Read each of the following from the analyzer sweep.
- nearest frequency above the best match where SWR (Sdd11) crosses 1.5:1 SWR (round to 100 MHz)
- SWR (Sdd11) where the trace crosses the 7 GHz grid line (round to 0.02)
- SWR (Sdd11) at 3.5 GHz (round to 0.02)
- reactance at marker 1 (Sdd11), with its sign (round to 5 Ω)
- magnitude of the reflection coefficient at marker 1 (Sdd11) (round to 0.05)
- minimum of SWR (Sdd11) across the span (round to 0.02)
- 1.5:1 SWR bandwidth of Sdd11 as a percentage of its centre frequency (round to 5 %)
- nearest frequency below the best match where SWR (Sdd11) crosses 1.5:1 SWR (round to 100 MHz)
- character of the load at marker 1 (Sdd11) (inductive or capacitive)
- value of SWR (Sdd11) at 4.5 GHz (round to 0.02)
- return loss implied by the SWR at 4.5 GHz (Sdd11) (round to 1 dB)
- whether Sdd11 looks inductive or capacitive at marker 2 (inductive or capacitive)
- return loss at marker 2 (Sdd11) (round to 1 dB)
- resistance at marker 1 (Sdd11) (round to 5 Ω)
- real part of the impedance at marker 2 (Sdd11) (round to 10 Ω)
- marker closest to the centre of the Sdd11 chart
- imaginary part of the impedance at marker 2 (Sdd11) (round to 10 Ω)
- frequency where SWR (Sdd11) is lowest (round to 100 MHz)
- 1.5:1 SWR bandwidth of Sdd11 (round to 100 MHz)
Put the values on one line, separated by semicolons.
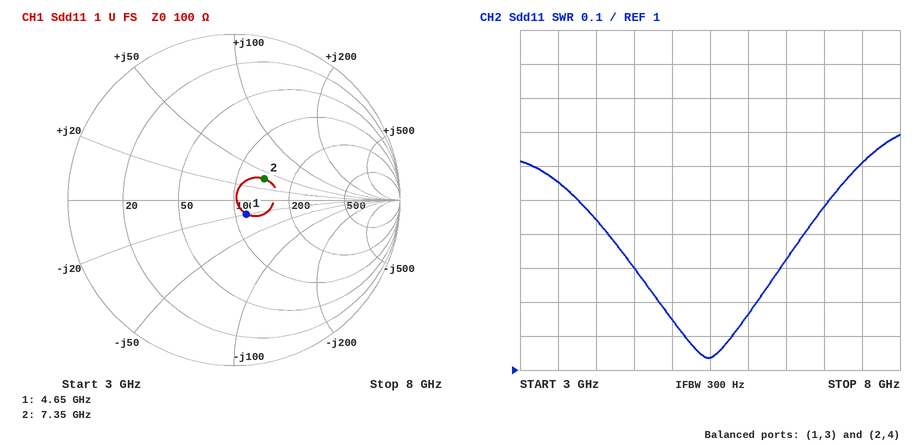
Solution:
7.1 GHz; 1.48; 1.56; -20 Ω; 0.10; 1.04; 60 %; 3.8 GHz; capacitive; 1.30; 18 dB; inductive; 13 dB; 115 Ω; 140 Ω; marker 1; +40 Ω; 5.5 GHz; 3.3 GHz
